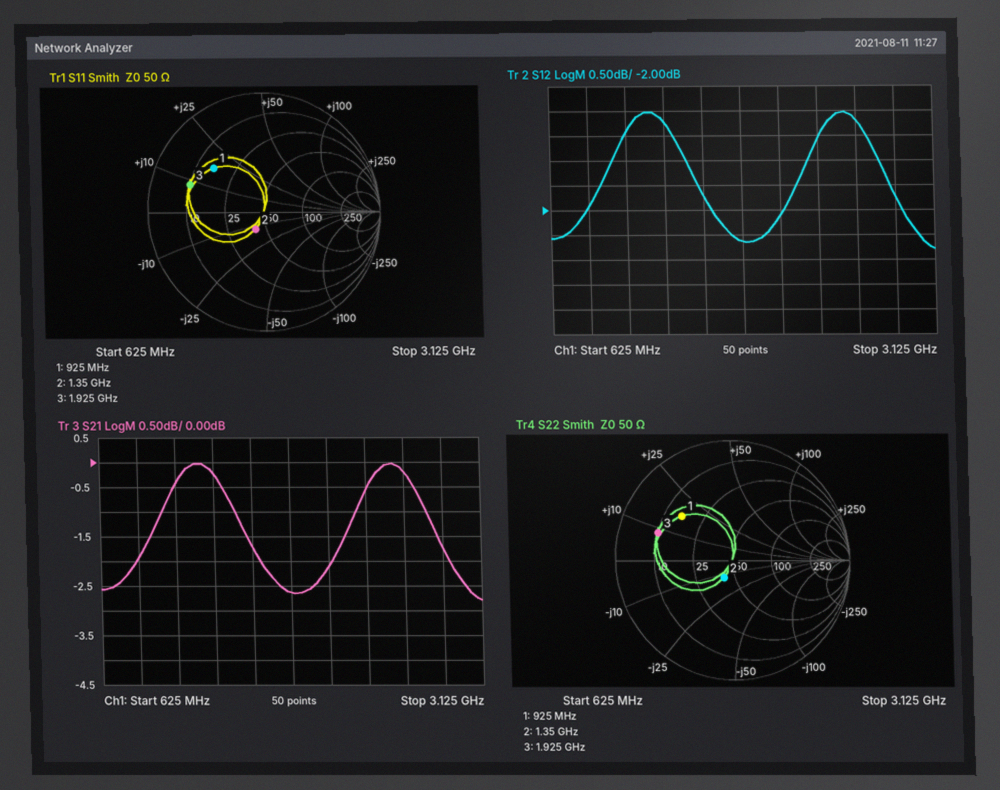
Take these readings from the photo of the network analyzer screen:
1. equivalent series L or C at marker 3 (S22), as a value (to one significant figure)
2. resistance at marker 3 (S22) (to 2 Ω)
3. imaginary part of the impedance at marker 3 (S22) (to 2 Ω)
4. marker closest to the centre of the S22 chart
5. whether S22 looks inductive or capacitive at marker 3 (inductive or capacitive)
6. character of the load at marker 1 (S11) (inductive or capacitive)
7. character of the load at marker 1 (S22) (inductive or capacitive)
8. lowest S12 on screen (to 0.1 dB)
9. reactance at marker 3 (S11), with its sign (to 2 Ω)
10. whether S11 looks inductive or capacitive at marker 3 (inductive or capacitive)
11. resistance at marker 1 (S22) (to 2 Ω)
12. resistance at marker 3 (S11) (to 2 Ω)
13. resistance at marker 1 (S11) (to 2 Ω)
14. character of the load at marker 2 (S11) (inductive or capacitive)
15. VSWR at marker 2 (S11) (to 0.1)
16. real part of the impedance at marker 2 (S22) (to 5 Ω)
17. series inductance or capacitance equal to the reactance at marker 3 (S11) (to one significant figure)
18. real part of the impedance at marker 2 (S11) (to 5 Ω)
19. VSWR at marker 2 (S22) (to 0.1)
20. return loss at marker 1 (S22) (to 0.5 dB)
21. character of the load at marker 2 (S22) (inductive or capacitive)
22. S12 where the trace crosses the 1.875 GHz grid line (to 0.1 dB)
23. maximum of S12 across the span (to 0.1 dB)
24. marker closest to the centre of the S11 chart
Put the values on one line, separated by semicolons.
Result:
700 pH; 10 Ω; +8 Ω; marker 2; inductive; inductive; inductive; -2.8 dB; +8 Ω; inductive; 16 Ω; 10 Ω; 16 Ω; capacitive; 1.4; 40 Ω; 700 pH; 40 Ω; 1.4; 5.0 dB; capacitive; -2.6 dB; 0.0 dB; marker 2
